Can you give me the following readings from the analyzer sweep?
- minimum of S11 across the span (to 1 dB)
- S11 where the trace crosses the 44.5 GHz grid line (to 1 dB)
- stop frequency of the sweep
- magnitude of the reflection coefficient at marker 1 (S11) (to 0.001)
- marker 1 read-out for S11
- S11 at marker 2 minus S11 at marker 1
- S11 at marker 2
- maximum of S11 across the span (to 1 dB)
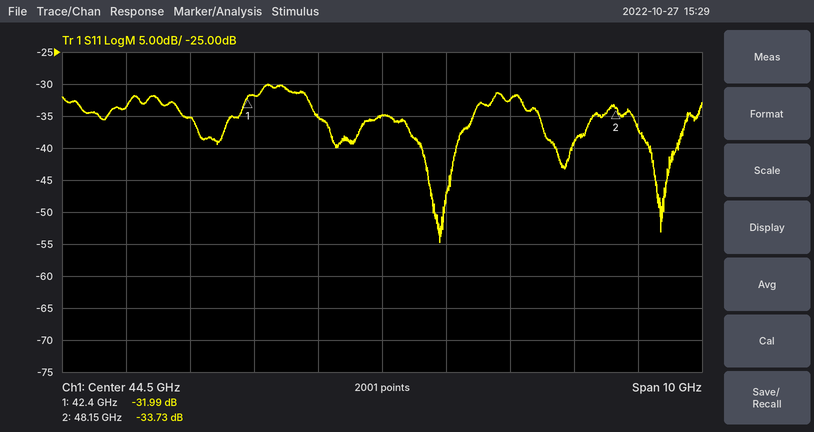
-55 dB
-35 dB
49.5 GHz
0.025
-31.99 dB
-1.74 dB
-33.73 dB
-30 dB
